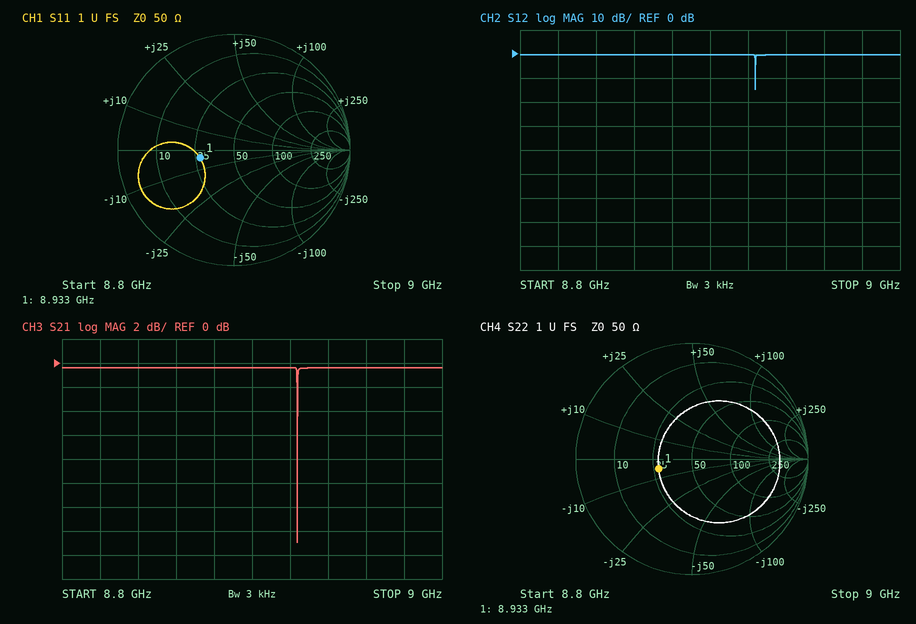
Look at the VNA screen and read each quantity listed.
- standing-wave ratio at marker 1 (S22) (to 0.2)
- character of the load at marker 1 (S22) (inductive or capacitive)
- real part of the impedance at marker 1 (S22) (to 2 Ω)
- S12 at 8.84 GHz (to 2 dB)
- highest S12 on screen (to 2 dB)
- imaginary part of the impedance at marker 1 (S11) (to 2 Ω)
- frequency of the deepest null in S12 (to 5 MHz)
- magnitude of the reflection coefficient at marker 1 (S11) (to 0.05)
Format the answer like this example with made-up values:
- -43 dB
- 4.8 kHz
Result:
- 1.8
- capacitive
- 28 Ω
- 0 dB
- 0 dB
- -4 Ω
- 8.925 GHz
- 0.30
